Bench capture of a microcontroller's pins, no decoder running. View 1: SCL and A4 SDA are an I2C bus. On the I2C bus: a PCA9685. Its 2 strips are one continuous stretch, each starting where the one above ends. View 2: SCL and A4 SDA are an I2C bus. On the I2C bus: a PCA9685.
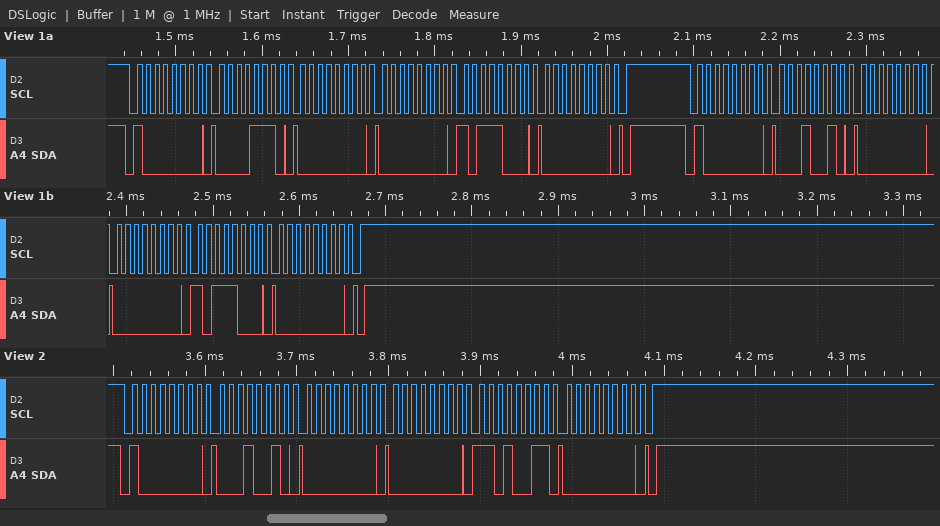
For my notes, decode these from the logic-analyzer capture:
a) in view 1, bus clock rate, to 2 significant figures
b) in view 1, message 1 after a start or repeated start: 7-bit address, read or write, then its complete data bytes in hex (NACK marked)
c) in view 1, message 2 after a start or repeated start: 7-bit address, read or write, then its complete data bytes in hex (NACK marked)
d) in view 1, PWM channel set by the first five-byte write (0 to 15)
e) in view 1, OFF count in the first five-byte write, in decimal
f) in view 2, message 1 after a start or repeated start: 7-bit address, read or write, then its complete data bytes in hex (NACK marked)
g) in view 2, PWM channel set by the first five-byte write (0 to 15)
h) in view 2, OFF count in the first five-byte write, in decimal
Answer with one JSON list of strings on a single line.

["100 kHz", "0x40 write: 0E 00 00 B8 00", "0x40 write: 12 00 00 B8 00", "2", "184", "0x40 write: 12 00 00 D3 00", "3", "211"]
